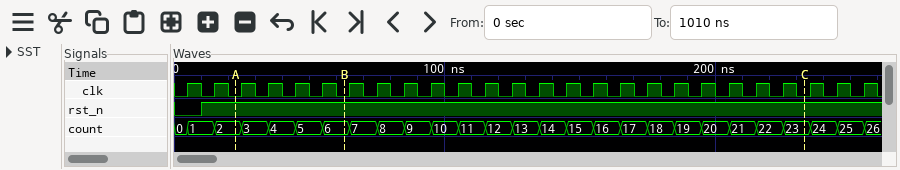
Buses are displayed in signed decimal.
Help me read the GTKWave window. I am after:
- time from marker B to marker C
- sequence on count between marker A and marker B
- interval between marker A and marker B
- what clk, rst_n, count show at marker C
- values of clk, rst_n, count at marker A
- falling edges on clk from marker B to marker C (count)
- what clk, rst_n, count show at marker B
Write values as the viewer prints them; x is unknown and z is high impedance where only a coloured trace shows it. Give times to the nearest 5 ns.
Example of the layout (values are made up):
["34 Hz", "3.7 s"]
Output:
["170 ns", "2, 3, 4, 5, 6", "40 ns", "clk=0, rst_n=1, count=23", "clk=0, rst_n=1, count=2", "17", "clk=0, rst_n=1, count=6"]
